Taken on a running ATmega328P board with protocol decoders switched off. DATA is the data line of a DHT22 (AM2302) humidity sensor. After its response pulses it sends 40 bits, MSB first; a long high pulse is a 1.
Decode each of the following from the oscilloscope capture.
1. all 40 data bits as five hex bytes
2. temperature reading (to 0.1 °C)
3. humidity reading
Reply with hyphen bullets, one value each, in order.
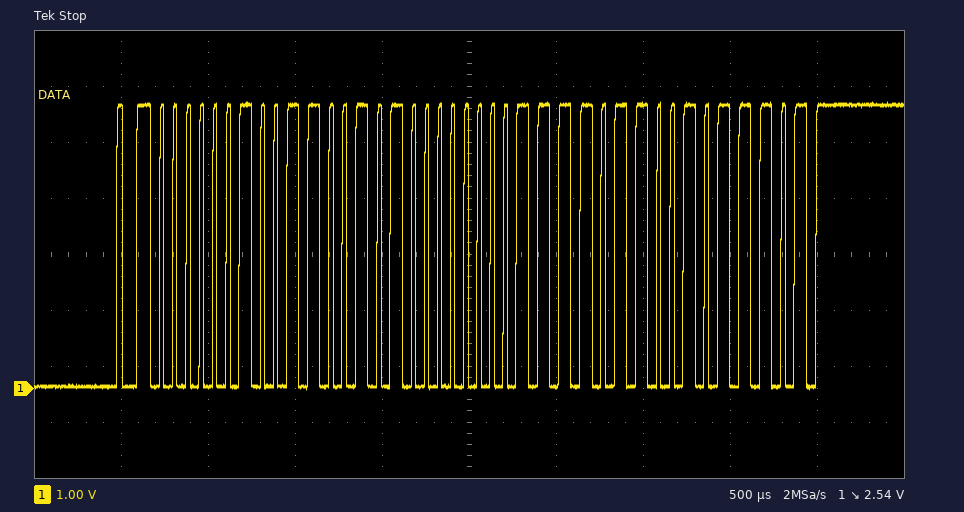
- 02 65 00 F6 5D
- 24.6 °C
- 61.3 %
